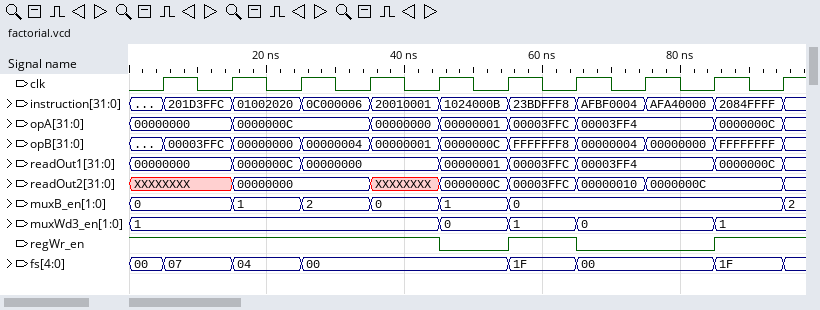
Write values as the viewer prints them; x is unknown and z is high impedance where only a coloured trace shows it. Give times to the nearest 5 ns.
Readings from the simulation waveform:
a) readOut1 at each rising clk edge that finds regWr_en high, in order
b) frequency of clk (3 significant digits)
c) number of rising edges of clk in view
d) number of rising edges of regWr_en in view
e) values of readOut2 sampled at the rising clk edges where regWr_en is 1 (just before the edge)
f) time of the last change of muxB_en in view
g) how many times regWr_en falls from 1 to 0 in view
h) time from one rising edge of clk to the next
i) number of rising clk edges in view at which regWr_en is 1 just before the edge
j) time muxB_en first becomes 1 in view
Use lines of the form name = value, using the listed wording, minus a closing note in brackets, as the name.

readOut1 at each rising clk edge that finds regWr_en high, in order = 00000000, 00000000, 0000000C, 00000000, 00000000, 00003FFC, 0000000C
frequency of clk = 100 MHz
number of rising edges of clk in view = 10
number of rising edges of regWr_en in view = 2
values of readOut2 sampled at the rising clk edges where regWr_en is 1 = XXXXXXXX, XXXXXXXX, 00000000, 00000000, XXXXXXXX, 00003FFC, 0000000C
time of the last change of muxB_en in view = 95 ns
how many times regWr_en falls from 1 to 0 in view = 2
time from one rising edge of clk to the next = 10 ns
number of rising clk edges in view at which regWr_en is 1 just before the edge = 7
time muxB_en first becomes 1 in view = 15 ns
